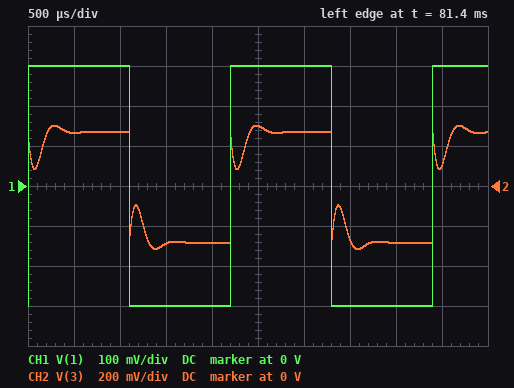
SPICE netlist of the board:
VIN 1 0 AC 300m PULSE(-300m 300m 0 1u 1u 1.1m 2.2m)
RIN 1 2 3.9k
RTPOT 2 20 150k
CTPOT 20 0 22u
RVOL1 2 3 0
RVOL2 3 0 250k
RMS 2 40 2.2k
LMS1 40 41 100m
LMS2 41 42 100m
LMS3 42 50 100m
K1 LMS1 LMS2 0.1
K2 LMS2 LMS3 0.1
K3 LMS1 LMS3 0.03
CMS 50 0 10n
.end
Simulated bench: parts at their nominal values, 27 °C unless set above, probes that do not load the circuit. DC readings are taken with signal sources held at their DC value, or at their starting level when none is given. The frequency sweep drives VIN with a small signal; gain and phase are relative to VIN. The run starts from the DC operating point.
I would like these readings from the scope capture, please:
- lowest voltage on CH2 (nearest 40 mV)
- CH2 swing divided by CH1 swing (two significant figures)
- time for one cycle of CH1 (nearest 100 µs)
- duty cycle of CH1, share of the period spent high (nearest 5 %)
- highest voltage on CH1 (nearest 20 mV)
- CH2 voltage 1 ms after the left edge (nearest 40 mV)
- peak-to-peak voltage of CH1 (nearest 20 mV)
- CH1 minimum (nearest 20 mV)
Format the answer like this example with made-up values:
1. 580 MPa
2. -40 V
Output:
1. -320 mV
2. 1.0
3. 2.2 ms
4. 50 %
5. 300 mV
6. 280 mV
7. 600 mV
8. -300 mV
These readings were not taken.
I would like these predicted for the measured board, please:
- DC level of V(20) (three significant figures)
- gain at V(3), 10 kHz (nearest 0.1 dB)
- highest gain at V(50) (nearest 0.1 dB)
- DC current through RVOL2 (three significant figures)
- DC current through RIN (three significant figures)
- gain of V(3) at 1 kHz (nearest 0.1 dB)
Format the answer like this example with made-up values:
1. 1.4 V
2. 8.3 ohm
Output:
1. -277 mV
2. -1.0 dB
3. 0.6 dB
4. 1.11 µA
5. 5.94 µA
6. -1.3 dB
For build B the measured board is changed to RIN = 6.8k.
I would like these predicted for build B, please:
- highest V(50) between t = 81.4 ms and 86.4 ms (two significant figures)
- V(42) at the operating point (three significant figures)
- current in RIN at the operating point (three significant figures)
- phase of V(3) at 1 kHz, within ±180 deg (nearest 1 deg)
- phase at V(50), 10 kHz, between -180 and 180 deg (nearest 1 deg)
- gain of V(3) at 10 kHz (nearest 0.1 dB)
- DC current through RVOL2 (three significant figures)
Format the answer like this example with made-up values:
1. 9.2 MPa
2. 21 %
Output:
1. 290 mV
2. -283 mV
3. 2.48 µA
4. -23 deg
5. -157 deg
6. -1.2 dB
7. 1.13 µA
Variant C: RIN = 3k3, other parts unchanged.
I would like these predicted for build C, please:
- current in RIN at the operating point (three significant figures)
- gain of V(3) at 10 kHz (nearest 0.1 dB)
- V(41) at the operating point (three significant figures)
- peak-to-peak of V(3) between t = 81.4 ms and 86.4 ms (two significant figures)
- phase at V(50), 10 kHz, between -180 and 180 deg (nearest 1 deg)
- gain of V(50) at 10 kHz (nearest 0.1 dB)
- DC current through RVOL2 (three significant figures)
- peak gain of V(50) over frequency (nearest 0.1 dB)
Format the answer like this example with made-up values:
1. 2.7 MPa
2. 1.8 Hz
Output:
1. 8.23 µA
2. 0.5 dB
3. -327 mV
4. 730 mV
5. -164 deg
6. -21.6 dB
7. 1.31 µA
8. 2.1 dB
